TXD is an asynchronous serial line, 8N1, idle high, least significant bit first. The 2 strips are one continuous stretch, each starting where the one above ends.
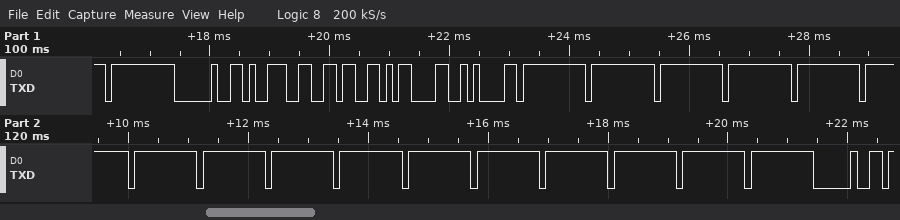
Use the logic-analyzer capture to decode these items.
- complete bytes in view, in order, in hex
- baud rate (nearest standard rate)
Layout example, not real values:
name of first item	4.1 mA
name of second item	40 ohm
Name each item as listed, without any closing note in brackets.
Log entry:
complete bytes in view, in order, in hex	FF 20 39 36 0D 0A FF FF FF FF FF FF FF FF FF FF FF FF FF FF FF FF 20
baud rate	9600 baud
